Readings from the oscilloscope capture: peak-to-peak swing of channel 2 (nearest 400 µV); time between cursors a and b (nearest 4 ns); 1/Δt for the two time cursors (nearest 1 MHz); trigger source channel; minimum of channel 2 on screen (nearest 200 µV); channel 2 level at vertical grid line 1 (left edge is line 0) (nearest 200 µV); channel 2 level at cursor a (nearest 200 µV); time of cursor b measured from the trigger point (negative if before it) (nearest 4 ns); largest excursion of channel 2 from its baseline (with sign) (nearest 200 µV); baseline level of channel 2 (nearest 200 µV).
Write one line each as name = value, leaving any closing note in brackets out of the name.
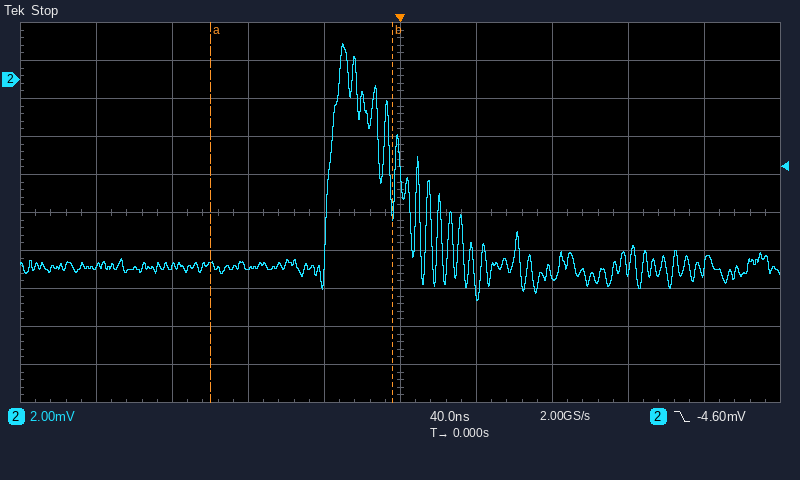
peak-to-peak swing of channel 2 = 13.6 mV
time between cursors a and b = 96 ns
1/Δt for the two time cursors = 10 MHz
trigger source channel = channel 2
minimum of channel 2 on screen = -11.6 mV
channel 2 level at vertical grid line 1 (left edge is line 0) = -9.8 mV
channel 2 level at cursor a = -9.8 mV
time of cursor b measured from the trigger point (negative if before it) = -4 ns
largest excursion of channel 2 from its baseline (with sign) = +11.8 mV
baseline level of channel 2 = -9.8 mV
